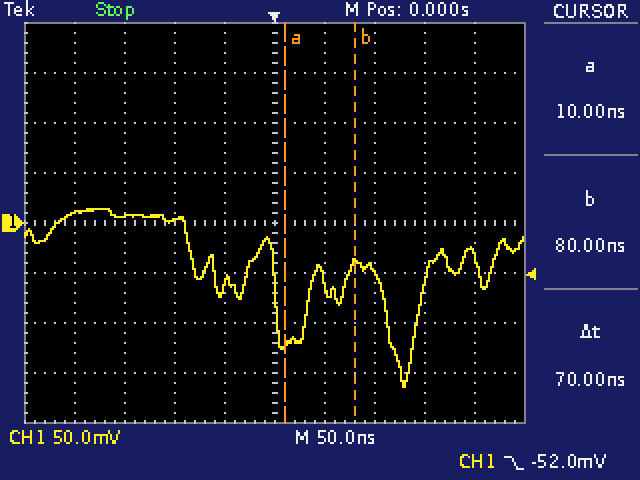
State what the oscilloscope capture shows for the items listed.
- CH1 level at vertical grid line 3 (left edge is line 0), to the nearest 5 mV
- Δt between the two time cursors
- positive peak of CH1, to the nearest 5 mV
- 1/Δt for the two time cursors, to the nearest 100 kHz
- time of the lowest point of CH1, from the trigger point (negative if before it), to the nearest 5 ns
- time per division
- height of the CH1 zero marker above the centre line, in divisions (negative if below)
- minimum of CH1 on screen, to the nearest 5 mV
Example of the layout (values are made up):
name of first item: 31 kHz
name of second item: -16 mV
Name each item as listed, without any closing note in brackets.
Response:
CH1 level at vertical grid line 3 (left edge is line 0), to the nearest 5 mV: 5 mV
Δt between the two time cursors: 70 ns
positive peak of CH1, to the nearest 5 mV: 15 mV
1/Δt for the two time cursors, to the nearest 100 kHz: 14.3 MHz
time of the lowest point of CH1, from the trigger point (negative if before it), to the nearest 5 ns: +130 ns
time per division: 50 ns
height of the CH1 zero marker above the centre line, in divisions: 0.0 div
minimum of CH1 on screen, to the nearest 5 mV: -165 mV
